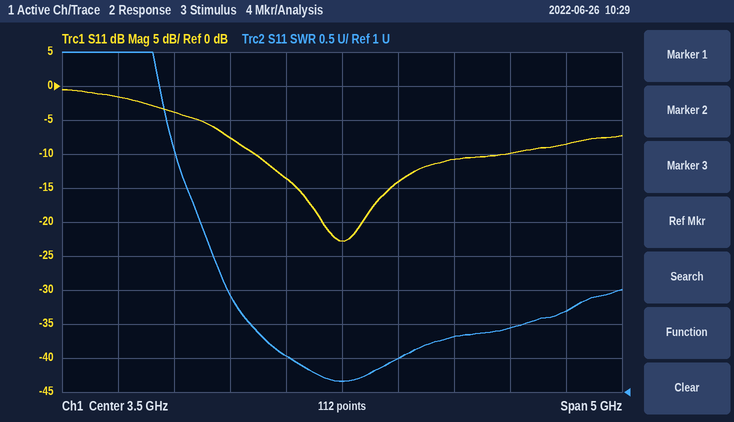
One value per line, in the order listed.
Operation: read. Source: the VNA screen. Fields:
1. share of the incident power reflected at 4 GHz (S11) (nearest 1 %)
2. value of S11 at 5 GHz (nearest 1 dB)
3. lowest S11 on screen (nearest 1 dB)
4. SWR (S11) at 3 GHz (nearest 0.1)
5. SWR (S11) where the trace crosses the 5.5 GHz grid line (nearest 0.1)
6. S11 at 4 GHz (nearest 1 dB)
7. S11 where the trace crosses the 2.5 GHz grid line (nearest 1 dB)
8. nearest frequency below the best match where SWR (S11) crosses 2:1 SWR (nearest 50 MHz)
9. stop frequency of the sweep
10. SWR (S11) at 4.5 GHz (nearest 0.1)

4 %
-10 dB
-23 dB
1.5
2.2
-14 dB
-8 dB
2.70 GHz
6 GHz
1.8
